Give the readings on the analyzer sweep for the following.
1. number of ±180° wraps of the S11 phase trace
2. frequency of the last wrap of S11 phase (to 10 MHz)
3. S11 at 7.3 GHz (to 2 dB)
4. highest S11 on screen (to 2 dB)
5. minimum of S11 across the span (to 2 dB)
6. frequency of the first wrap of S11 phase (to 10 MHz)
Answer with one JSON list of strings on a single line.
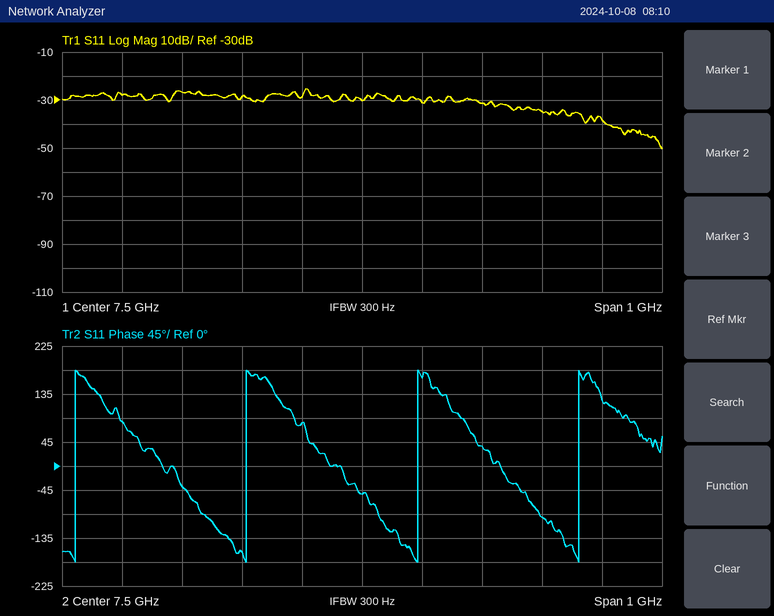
["4", "7.86 GHz", "-28 dB", "-26 dB", "-50 dB", "7.02 GHz"]
